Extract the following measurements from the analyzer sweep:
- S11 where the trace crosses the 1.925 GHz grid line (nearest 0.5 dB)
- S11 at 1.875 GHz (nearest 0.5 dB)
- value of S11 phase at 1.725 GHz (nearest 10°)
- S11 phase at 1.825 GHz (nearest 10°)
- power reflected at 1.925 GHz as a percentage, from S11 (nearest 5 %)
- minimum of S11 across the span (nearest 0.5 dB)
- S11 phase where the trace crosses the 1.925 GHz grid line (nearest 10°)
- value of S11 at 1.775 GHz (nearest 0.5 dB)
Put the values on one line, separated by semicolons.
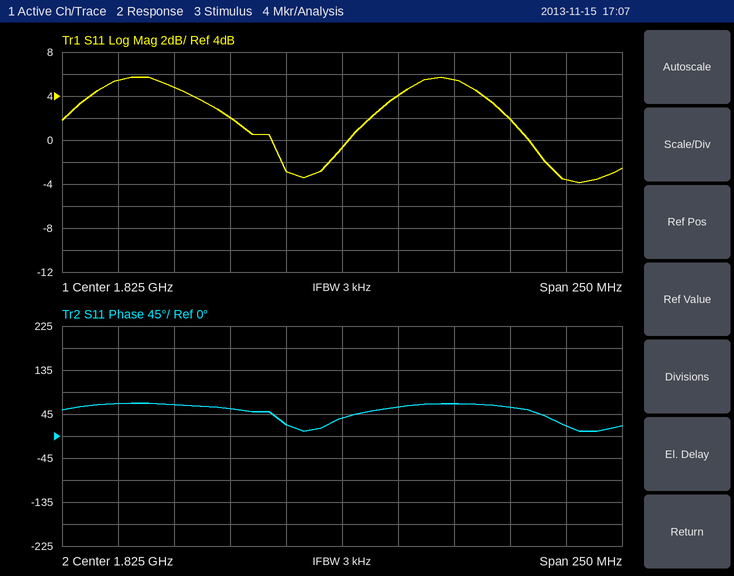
-3.5 dB; 5.5 dB; 70°; 40°; 45 %; -4.0 dB; 20°; 2.0 dB
